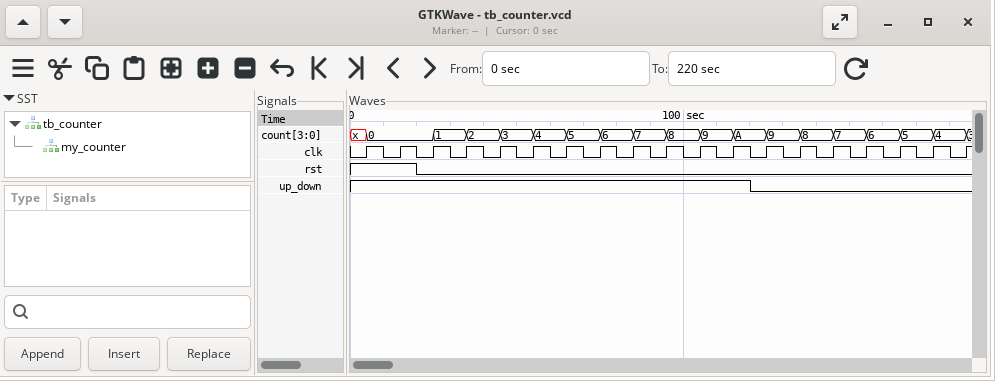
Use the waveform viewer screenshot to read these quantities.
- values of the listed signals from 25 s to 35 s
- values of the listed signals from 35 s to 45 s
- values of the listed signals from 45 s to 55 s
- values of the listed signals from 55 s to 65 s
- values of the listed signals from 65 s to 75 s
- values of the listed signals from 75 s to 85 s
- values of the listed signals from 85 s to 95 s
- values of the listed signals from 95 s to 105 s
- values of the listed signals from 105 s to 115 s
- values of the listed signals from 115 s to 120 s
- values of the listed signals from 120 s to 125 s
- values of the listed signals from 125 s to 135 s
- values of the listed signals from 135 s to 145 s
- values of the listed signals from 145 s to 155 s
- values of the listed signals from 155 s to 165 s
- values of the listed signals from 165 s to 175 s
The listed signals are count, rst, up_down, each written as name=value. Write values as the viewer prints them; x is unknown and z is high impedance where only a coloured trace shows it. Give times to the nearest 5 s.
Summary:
count=1, rst=0, up_down=1
count=2, rst=0, up_down=1
count=3, rst=0, up_down=1
count=4, rst=0, up_down=1
count=5, rst=0, up_down=1
count=6, rst=0, up_down=1
count=7, rst=0, up_down=1
count=8, rst=0, up_down=1
count=9, rst=0, up_down=1
count=A, rst=0, up_down=1
count=A, rst=0, up_down=0
count=9, rst=0, up_down=0
count=8, rst=0, up_down=0
count=7, rst=0, up_down=0
count=6, rst=0, up_down=0
count=5, rst=0, up_down=0
